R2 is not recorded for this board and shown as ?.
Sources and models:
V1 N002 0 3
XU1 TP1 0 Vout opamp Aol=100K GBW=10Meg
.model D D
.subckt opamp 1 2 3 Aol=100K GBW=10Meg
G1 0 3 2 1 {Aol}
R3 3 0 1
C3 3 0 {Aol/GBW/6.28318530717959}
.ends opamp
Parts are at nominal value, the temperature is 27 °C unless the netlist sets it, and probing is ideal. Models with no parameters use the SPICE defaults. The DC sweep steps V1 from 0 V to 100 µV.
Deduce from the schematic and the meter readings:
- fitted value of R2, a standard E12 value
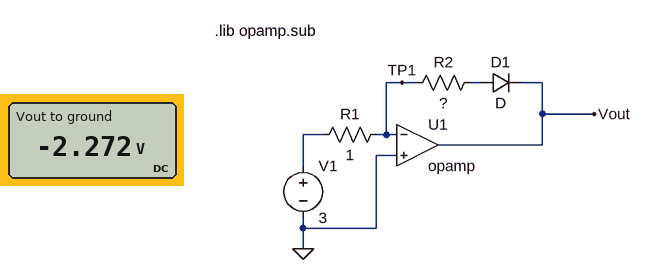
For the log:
0.47 Ω
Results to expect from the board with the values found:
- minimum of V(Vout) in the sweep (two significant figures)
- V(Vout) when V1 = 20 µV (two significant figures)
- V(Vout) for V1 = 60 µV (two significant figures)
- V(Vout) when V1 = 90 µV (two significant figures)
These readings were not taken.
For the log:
-590 mV
-550 mV
-580 mV
-590 mV
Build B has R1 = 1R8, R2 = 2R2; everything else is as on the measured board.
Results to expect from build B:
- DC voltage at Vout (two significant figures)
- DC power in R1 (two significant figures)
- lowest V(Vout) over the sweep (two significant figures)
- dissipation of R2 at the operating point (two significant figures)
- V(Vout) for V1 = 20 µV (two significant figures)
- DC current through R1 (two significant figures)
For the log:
-4.5 V
5.0 W
-580 mV
6.1 W
-530 mV
1.7 A
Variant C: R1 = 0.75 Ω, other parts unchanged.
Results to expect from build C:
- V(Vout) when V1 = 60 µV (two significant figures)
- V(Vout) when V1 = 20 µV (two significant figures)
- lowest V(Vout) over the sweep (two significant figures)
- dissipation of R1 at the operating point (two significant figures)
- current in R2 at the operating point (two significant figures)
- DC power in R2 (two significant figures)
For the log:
-590 mV
-550 mV
-600 mV
12 W
4.0 A
7.5 W
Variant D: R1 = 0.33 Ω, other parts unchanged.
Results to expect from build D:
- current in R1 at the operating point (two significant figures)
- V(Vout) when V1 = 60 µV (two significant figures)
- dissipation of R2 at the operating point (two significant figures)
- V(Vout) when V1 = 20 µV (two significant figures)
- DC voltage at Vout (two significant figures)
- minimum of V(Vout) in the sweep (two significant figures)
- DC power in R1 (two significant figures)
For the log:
9.1 A
-610 mV
39 W
-570 mV
-5.2 V
-620 mV
27 W
